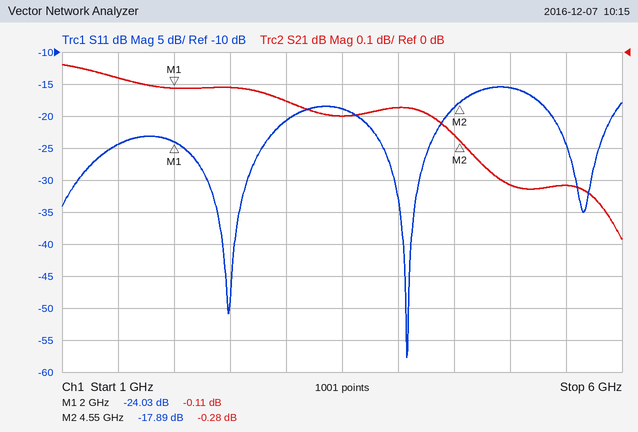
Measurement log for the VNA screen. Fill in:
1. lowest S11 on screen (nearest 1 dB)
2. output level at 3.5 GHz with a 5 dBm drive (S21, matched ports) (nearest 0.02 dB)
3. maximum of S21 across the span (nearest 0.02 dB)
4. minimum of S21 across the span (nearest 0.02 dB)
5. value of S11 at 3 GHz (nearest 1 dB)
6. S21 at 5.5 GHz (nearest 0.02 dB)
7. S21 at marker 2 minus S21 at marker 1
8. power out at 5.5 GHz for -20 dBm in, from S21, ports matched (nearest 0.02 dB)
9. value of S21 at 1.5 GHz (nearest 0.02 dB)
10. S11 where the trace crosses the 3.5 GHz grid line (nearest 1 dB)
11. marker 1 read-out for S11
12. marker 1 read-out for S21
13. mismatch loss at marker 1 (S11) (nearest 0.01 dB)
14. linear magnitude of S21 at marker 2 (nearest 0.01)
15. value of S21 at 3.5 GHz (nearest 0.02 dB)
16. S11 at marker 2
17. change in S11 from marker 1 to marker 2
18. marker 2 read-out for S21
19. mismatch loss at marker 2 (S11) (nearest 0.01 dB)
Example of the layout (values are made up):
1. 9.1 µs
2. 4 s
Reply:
1. -58 dB
2. 4.80 dBm
3. -0.04 dB
4. -0.58 dB
5. -21 dB
6. -0.42 dB
7. -0.17 dB
8. -20.42 dBm
9. -0.08 dB
10. -19 dB
11. -24.03 dB
12. -0.11 dB
13. 0.02 dB
14. 0.97
15. -0.20 dB
16. -17.89 dB
17. 6.14 dB
18. -0.28 dB
19. 0.07 dB
